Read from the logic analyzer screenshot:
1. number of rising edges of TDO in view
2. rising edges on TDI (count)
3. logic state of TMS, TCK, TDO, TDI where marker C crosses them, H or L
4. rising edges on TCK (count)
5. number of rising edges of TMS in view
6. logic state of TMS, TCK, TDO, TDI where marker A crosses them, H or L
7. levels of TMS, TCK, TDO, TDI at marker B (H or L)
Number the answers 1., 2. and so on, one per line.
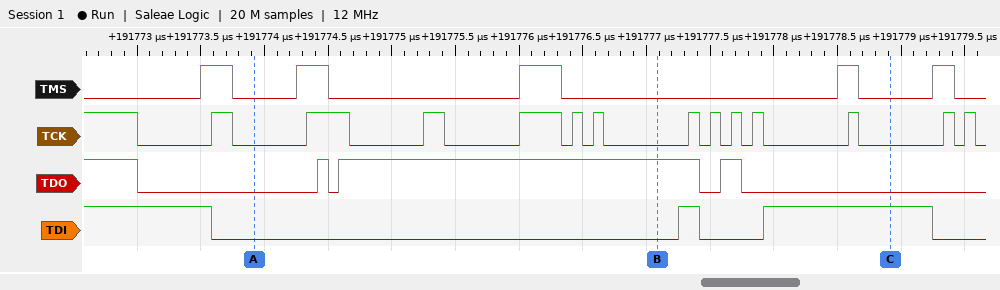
1. 3
2. 2
3. TMS=L, TCK=L, TDO=L, TDI=H
4. 13
5. 5
6. TMS=L, TCK=L, TDO=L, TDI=L
7. TMS=L, TCK=L, TDO=H, TDI=L
